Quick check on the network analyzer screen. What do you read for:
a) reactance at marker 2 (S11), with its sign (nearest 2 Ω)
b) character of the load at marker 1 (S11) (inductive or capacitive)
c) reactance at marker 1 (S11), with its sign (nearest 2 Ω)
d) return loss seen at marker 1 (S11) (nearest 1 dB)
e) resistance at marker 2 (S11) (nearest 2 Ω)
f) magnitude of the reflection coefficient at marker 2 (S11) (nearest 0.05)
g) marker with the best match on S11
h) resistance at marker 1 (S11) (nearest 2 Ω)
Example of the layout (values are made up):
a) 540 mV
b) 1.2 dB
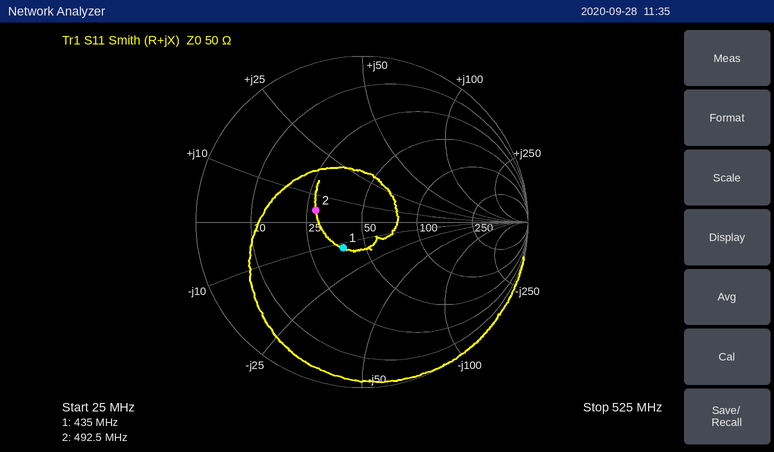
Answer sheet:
a) +4 Ω
b) capacitive
c) -12 Ω
d) 14 dB
e) 28 Ω
f) 0.30
g) marker 1
h) 38 Ω
